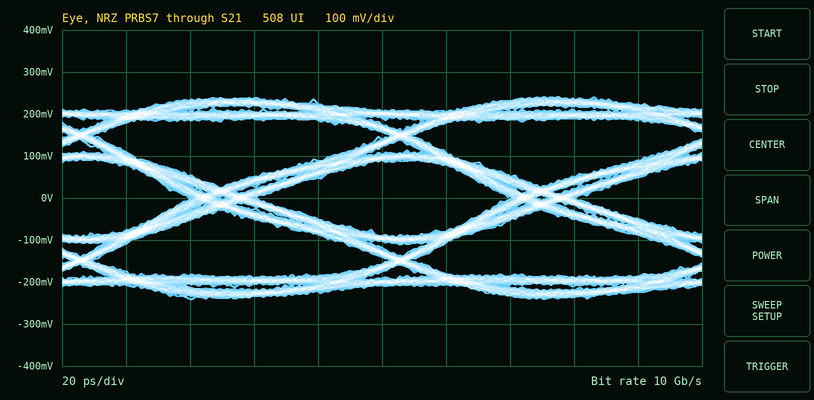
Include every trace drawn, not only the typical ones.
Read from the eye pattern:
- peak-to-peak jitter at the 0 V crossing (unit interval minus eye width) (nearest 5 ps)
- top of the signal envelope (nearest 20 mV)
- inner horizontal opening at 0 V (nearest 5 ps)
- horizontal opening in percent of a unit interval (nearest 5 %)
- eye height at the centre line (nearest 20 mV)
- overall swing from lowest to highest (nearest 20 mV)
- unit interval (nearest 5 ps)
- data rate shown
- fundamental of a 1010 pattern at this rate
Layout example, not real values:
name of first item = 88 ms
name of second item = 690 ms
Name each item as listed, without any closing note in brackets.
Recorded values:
peak-to-peak jitter at the 0 V crossing (unit interval minus eye width) = 20 ps
top of the signal envelope = 240 mV
inner horizontal opening at 0 V = 80 ps
horizontal opening in percent of a unit interval = 80 %
eye height at the centre line = 180 mV
overall swing from lowest to highest = 480 mV
unit interval = 100 ps
data rate shown = 10 Gb/s
fundamental of a 1010 pattern at this rate = 5 GHz
